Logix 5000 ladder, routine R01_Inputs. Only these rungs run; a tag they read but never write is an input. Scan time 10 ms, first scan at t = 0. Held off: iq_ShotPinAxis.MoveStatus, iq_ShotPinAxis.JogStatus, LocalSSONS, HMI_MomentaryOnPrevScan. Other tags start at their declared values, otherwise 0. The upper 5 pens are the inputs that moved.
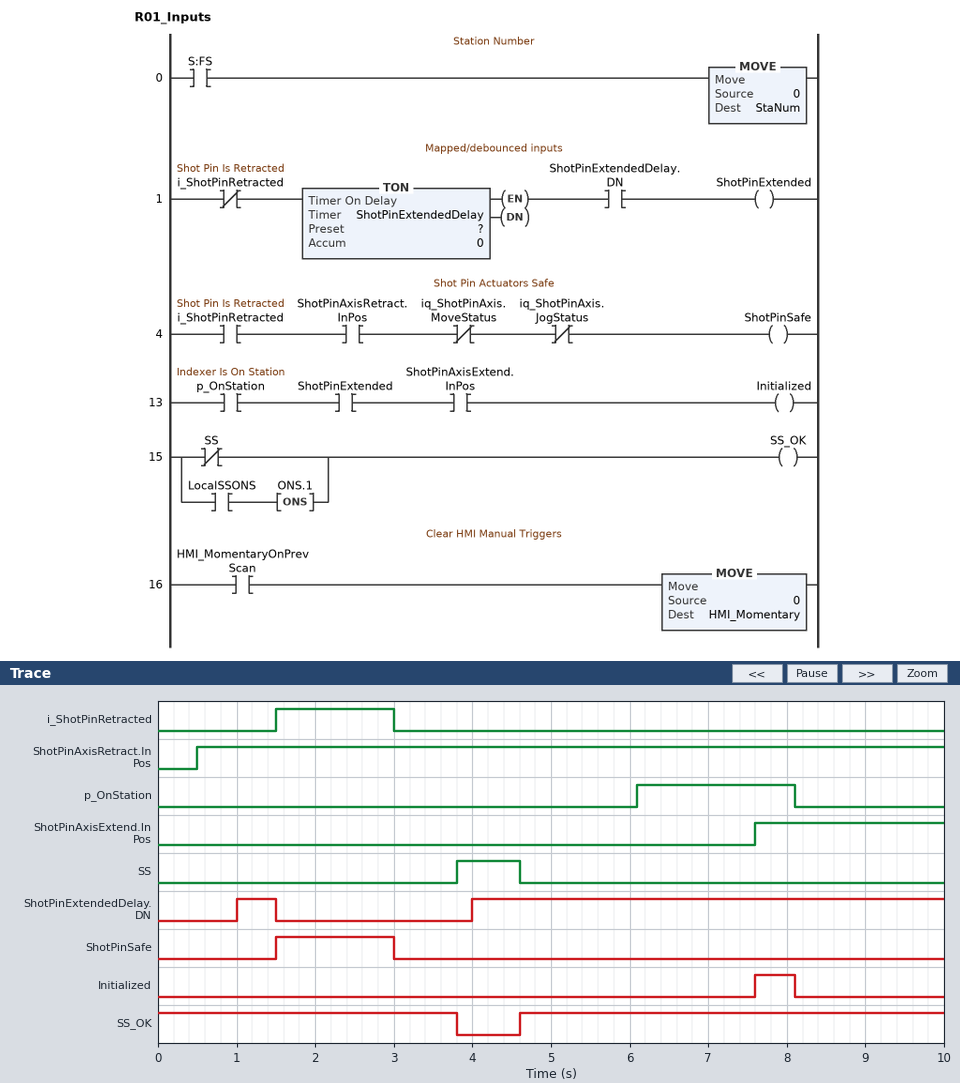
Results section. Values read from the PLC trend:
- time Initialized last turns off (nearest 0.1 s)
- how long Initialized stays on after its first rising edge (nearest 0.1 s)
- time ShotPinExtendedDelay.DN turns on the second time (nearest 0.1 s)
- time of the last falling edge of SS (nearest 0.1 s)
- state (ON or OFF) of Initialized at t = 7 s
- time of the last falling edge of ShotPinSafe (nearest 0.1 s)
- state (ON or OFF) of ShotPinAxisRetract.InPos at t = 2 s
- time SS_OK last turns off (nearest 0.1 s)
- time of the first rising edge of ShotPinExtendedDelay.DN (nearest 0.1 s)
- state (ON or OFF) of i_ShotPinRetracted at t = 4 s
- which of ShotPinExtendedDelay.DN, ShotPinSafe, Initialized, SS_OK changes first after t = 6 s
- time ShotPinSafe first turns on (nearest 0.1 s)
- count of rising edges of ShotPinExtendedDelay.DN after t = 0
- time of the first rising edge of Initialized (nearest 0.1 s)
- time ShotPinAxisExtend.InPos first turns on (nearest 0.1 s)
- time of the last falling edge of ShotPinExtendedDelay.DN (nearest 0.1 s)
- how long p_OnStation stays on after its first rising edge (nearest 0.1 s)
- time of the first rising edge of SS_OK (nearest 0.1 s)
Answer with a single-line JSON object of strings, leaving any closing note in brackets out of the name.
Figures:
{"time Initialized last turns off": "8.1 s", "how long Initialized stays on after its first rising edge": "0.5 s", "time ShotPinExtendedDelay.DN turns on the second time": "4.0 s", "time of the last falling edge of SS": "4.6 s", "state (ON or OFF) of Initialized at t = 7 s": "OFF", "time of the last falling edge of ShotPinSafe": "3.0 s", "state (ON or OFF) of ShotPinAxisRetract.InPos at t = 2 s": "ON", "time SS_OK last turns off": "3.8 s", "time of the first rising edge of ShotPinExtendedDelay.DN": "1.0 s", "state (ON or OFF) of i_ShotPinRetracted at t = 4 s": "OFF", "which of ShotPinExtendedDelay.DN, ShotPinSafe, Initialized, SS_OK changes first after t = 6 s": "Initialized", "time ShotPinSafe first turns on": "1.5 s", "count of rising edges of ShotPinExtendedDelay.DN after t = 0": "2", "time of the first rising edge of Initialized": "7.6 s", "time ShotPinAxisExtend.InPos first turns on": "7.6 s", "time of the last falling edge of ShotPinExtendedDelay.DN": "1.5 s", "how long p_OnStation stays on after its first rising edge": "2.0 s", "time of the first rising edge of SS_OK": "4.6 s"}
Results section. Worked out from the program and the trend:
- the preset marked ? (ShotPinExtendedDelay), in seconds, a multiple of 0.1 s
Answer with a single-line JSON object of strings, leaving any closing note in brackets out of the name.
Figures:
{"the preset marked ? (ShotPinExtendedDelay), in seconds, a multiple of 0.1 s": "1.0 s"}
